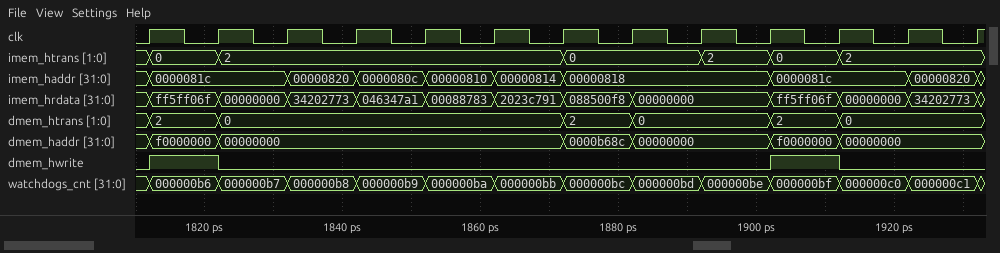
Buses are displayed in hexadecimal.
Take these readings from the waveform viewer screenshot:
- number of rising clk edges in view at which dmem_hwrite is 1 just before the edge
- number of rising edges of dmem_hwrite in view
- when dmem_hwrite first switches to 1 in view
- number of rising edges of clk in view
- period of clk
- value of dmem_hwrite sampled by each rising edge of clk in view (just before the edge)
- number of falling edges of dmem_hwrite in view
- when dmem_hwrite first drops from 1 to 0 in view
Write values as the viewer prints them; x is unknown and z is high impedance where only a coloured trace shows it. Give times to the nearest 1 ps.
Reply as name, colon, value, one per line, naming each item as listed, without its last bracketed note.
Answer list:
number of rising clk edges in view at which dmem_hwrite is 1 just before the edge: 2
number of rising edges of dmem_hwrite in view: 2
when dmem_hwrite first switches to 1 in view: 1812 ps
number of rising edges of clk in view: 13
period of clk: 10 ps
value of dmem_hwrite sampled by each rising edge of clk in view: 0 1 0 0 0 0 0 0 0 0 1 0 0
number of falling edges of dmem_hwrite in view: 2
when dmem_hwrite first drops from 1 to 0 in view: 1822 ps
